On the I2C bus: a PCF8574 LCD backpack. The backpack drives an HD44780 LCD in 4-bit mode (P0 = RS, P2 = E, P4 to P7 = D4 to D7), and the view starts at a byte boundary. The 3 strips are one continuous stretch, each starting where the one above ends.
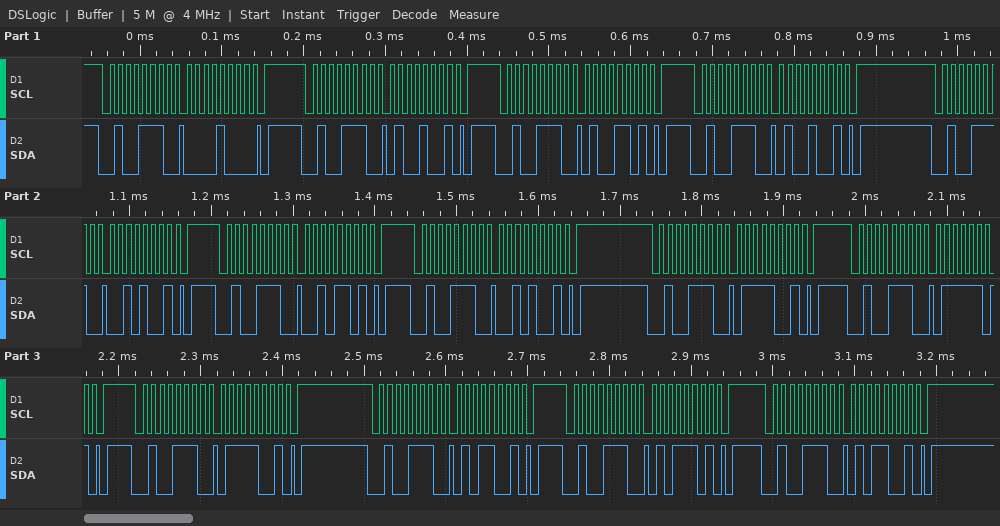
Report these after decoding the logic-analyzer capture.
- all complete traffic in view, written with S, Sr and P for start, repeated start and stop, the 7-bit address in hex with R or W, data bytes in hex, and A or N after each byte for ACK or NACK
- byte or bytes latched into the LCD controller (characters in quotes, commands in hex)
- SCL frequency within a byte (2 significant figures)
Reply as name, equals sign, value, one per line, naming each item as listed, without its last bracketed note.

all complete traffic in view, written with S, Sr and P for start, repeated start and stop, the 7-bit address in hex with R or W, data bytes in hex, and A or N after each byte for ACK or NACK = S 27W A 08 A P S 27W A 49 A P S 27W A 4D A P S 27W A 49 A P S 27W A 29 A P S 27W A 2D A P S 27W A 29 A P S 27W A 79 A P S 27W A 7D A P S 27W A 79 A P S 27W A 59 A P S 27W A 5D A P S 27W A 59 A P
byte or bytes latched into the LCD controller = 'B' 'u'
SCL frequency within a byte = 100 kHz
